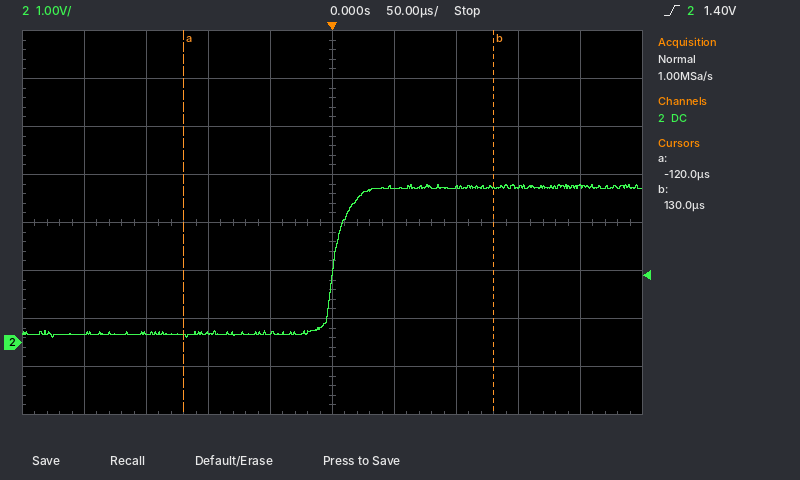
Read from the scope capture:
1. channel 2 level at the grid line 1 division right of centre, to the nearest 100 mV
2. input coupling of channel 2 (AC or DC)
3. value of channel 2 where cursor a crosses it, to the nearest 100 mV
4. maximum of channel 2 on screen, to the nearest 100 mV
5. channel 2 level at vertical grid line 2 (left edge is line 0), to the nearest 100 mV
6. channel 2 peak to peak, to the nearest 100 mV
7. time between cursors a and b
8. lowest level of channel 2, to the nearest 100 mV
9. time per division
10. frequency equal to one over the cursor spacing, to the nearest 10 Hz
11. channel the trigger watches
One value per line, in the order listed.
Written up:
3.2 V
DC
100 mV
3.3 V
200 mV
3.2 V
250 µs
100 mV
50 µs
4.00 kHz
channel 2
